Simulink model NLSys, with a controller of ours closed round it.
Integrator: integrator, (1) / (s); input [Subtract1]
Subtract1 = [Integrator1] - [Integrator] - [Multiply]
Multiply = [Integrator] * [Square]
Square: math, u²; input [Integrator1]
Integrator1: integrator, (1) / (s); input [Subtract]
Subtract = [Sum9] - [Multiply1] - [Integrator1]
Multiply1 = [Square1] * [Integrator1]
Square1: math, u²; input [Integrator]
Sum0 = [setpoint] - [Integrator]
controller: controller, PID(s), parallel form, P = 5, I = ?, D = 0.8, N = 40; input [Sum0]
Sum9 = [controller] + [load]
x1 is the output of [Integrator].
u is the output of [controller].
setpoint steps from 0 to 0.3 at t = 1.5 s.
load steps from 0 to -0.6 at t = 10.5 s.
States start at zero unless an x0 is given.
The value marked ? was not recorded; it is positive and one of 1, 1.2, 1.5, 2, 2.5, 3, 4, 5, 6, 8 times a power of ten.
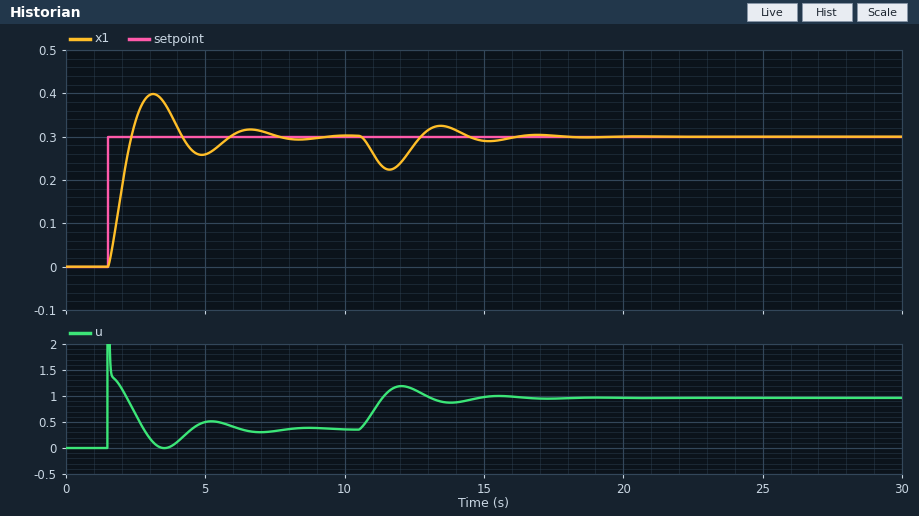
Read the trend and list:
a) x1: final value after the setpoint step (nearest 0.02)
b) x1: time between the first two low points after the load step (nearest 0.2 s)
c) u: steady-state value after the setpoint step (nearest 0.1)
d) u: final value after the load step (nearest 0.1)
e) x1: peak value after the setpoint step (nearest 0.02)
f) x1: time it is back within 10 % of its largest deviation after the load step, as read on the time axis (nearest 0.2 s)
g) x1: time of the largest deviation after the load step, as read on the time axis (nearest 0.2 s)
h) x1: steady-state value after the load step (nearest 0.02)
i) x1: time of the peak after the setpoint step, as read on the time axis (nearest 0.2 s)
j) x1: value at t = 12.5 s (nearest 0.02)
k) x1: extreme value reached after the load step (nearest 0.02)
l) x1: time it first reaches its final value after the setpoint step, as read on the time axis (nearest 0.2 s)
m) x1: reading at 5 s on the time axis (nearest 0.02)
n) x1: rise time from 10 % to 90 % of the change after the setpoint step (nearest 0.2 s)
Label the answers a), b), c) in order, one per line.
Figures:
a) 0.30
b) 3.6 s
c) 0.4
d) 1.0
e) 0.40
f) 15.6 s
g) 11.6 s
h) 0.30
i) 3.2 s
j) 0.28
k) 0.22
l) 2.4 s
m) 0.26
n) 0.6 s
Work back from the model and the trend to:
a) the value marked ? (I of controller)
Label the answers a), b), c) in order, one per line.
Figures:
a) 8
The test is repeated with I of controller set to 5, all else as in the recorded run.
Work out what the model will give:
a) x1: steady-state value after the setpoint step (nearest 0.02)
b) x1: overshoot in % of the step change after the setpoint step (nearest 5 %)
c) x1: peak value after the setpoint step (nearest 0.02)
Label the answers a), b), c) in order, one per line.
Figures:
a) 0.30
b) 20 %
c) 0.36
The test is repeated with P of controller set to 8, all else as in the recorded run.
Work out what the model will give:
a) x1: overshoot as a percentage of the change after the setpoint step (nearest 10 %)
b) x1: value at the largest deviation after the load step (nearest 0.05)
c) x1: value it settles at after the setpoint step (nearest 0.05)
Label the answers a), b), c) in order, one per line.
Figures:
a) 30 %
b) 0.25
c) 0.30
